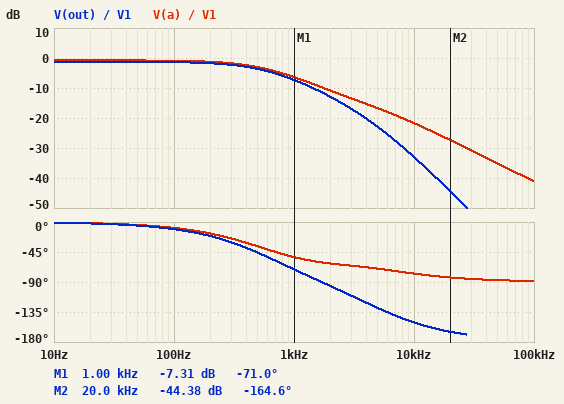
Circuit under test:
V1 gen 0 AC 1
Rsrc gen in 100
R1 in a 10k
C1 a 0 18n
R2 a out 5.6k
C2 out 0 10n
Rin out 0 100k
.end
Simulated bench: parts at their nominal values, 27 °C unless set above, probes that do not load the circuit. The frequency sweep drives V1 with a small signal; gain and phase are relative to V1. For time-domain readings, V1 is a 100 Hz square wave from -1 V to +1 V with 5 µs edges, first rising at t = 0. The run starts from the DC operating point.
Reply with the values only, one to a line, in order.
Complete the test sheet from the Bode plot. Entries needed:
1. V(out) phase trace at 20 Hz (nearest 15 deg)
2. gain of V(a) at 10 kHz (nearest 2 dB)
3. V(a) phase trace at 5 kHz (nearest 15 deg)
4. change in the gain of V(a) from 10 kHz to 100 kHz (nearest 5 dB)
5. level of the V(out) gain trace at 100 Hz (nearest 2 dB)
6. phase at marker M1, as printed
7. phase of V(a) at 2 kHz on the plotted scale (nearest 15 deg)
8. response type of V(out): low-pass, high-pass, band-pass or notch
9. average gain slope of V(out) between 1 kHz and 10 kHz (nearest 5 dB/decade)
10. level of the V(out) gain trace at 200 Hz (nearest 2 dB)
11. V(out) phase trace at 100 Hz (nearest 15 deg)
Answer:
0 deg
-22 dB
-75 deg
-20 dB
-2 dB
-71.0 deg
-60 deg
low-pass
-25 dB/decade
-2 dB
-15 deg
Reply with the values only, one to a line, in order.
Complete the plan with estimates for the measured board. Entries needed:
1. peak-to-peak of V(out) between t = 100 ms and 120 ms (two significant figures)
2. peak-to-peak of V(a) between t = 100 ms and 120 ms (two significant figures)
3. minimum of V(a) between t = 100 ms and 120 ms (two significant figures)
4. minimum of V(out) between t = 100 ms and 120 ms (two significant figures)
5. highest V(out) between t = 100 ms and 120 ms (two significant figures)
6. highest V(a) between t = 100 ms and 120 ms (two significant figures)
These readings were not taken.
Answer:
1.7 V
1.8 V
-910 mV
-860 mV
860 mV
910 mV
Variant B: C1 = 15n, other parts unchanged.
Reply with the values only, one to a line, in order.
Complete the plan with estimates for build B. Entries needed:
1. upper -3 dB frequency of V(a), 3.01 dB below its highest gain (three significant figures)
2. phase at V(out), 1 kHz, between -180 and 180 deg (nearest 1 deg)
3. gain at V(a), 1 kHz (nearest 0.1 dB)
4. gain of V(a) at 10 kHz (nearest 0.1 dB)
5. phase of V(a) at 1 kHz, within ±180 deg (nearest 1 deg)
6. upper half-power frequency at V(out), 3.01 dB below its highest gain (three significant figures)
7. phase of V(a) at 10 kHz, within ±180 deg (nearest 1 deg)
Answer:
674 Hz
-68 deg
-5.7 dB
-20.3 dB
-49 deg
643 Hz
-75 deg
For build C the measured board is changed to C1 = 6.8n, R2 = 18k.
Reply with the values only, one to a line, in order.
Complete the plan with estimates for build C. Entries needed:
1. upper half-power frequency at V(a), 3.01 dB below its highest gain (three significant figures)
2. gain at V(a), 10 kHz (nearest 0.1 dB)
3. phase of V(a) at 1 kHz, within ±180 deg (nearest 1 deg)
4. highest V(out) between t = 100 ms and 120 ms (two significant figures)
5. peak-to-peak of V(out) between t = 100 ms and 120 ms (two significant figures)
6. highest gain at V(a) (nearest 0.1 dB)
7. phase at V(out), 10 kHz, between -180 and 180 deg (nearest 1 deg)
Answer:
1.16 kHz
-13.3 dB
-27 deg
780 mV
1.6 V
-0.7 dB
-154 deg
